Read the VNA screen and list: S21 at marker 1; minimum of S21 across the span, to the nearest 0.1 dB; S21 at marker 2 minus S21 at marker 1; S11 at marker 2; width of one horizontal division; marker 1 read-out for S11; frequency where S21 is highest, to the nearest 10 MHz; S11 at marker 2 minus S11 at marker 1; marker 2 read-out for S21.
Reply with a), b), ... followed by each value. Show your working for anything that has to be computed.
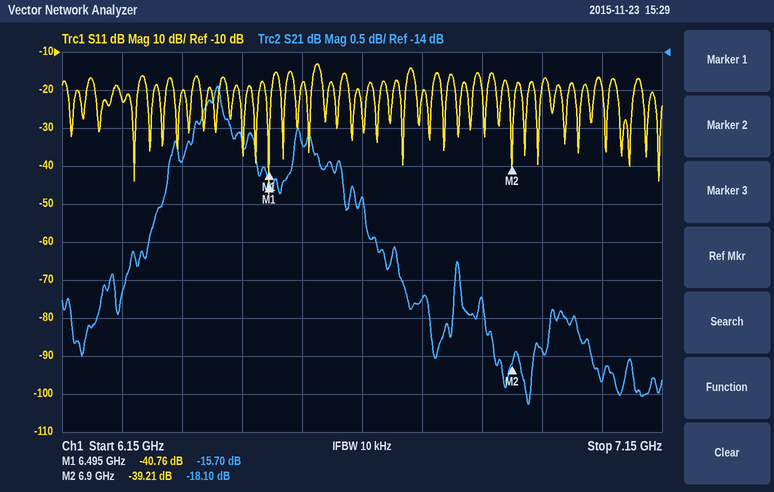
a) -15.70 dB
b) -18.6 dB
c) -18.1 − (-15.7) = -2.40 dB
d) -39.21 dB
e) 100 MHz
f) -40.76 dB
g) 6.41 GHz
h) -39.21 − (-40.76) = 1.55 dB
i) -18.10 dB
